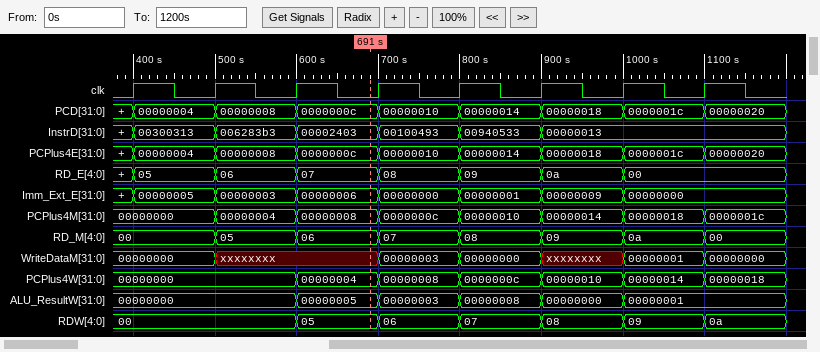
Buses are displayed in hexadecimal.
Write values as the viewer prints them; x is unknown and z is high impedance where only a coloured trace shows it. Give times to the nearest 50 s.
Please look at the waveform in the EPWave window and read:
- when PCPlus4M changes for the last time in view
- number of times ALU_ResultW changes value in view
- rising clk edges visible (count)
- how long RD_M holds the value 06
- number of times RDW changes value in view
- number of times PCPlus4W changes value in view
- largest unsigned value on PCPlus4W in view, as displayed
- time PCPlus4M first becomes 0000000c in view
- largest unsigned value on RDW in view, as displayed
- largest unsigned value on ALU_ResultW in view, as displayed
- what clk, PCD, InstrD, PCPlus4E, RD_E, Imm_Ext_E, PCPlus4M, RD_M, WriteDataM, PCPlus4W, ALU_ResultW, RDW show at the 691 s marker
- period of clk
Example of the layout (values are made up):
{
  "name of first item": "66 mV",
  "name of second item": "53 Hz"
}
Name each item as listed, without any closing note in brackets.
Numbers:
{
  "when PCPlus4M changes for the last time in view": "1100 s",
  "number of times ALU_ResultW changes value in view": "5",
  "rising clk edges visible": "8",
  "how long RD_M holds the value 06": "100 s",
  "number of times RDW changes value in view": "6",
  "number of times PCPlus4W changes value in view": "6",
  "largest unsigned value on PCPlus4W in view, as displayed": "00000018",
  "time PCPlus4M first becomes 0000000c in view": "700 s",
  "largest unsigned value on RDW in view, as displayed": "0a",
  "largest unsigned value on ALU_ResultW in view, as displayed": "00000008",
  "what clk, PCD, InstrD, PCPlus4E, RD_E, Imm_Ext_E, PCPlus4M, RD_M, WriteDataM, PCPlus4W, ALU_ResultW, RDW show at the 691 s marker": "clk=0, PCD=0000000c, InstrD=00002403, PCPlus4E=0000000c, RD_E=07, Imm_Ext_E=00000006, PCPlus4M=00000008, RD_M=06, WriteDataM=xxxxxxxx, PCPlus4W=00000004, ALU_ResultW=00000005, RDW=05",
  "period of clk": "100 s"
}
